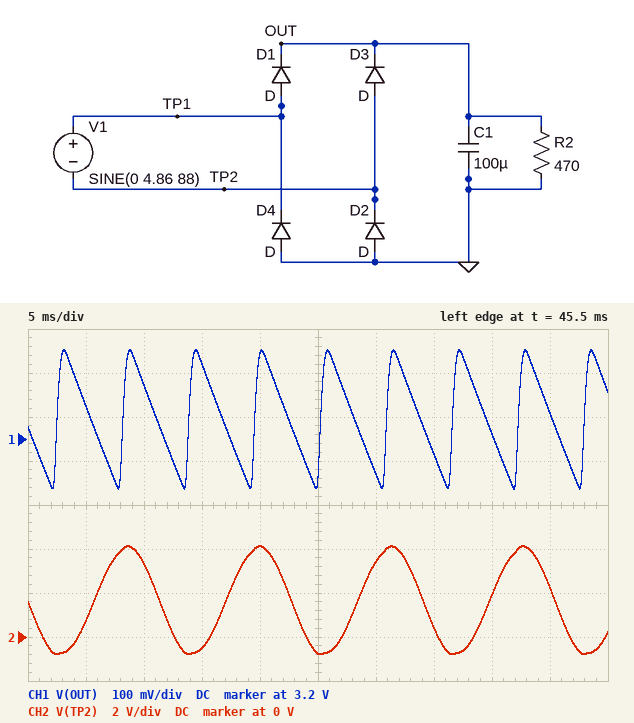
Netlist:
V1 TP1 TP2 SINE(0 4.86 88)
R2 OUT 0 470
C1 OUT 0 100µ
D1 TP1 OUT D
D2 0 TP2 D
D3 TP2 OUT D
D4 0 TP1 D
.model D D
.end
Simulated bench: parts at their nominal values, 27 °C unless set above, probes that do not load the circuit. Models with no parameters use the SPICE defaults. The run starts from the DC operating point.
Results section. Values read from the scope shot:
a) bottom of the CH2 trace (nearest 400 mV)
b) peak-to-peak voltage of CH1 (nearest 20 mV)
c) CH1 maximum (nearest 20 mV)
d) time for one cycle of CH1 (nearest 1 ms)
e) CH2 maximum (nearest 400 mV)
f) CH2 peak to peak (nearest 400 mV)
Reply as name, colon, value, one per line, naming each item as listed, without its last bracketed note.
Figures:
bottom of the CH2 trace: -800 mV
peak-to-peak voltage of CH1: 320 mV
CH1 maximum: 3.40 V
time for one cycle of CH1: 6 ms
CH2 maximum: 4.0 V
CH2 peak to peak: 4.8 V
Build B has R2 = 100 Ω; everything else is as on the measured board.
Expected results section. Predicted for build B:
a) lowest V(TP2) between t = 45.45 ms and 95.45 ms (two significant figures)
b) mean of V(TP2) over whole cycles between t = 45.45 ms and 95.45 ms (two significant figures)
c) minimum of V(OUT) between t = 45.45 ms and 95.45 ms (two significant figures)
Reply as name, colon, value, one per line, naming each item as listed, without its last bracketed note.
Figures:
lowest V(TP2) between t = 45.45 ms and 95.45 ms: -790 mV
mean of V(TP2) over whole cycles between t = 45.45 ms and 95.45 ms: 1.4 V
minimum of V(OUT) between t = 45.45 ms and 95.45 ms: 2.2 V
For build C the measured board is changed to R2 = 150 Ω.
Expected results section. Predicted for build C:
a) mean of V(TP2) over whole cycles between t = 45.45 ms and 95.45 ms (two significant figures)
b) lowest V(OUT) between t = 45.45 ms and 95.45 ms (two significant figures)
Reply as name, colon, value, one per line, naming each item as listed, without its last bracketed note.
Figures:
mean of V(TP2) over whole cycles between t = 45.45 ms and 95.45 ms: 1.5 V
lowest V(OUT) between t = 45.45 ms and 95.45 ms: 2.5 V
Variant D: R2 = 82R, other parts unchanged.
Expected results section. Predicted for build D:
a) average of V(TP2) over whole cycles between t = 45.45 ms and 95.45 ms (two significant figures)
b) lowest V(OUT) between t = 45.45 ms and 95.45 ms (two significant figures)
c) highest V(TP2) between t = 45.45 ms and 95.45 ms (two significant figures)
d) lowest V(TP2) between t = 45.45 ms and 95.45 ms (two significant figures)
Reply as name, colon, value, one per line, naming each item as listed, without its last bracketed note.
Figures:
average of V(TP2) over whole cycles between t = 45.45 ms and 95.45 ms: 1.4 V
lowest V(OUT) between t = 45.45 ms and 95.45 ms: 2.1 V
highest V(TP2) between t = 45.45 ms and 95.45 ms: 4.1 V
lowest V(TP2) between t = 45.45 ms and 95.45 ms: -790 mV
